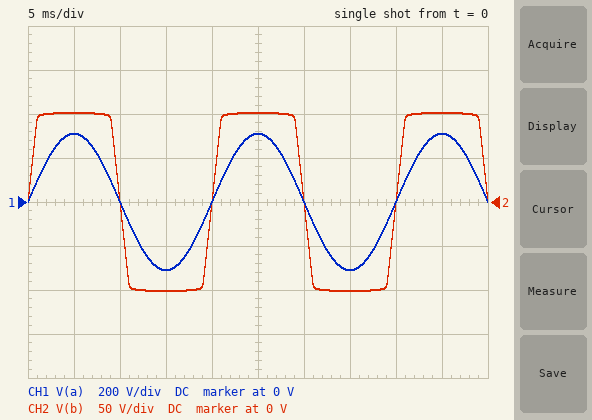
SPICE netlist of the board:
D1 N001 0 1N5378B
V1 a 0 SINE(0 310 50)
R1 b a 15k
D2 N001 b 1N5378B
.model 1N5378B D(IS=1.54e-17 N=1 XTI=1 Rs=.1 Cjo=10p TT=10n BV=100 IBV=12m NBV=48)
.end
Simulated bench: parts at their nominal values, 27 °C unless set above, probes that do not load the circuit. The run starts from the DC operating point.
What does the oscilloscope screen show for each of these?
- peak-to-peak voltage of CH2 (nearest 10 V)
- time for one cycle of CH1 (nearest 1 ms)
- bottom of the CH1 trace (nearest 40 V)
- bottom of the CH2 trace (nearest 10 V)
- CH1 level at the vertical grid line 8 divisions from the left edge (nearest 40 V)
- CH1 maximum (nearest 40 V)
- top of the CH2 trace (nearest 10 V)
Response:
200 V
20 ms
-320 V
-100 V
0 V
320 V
100 V
